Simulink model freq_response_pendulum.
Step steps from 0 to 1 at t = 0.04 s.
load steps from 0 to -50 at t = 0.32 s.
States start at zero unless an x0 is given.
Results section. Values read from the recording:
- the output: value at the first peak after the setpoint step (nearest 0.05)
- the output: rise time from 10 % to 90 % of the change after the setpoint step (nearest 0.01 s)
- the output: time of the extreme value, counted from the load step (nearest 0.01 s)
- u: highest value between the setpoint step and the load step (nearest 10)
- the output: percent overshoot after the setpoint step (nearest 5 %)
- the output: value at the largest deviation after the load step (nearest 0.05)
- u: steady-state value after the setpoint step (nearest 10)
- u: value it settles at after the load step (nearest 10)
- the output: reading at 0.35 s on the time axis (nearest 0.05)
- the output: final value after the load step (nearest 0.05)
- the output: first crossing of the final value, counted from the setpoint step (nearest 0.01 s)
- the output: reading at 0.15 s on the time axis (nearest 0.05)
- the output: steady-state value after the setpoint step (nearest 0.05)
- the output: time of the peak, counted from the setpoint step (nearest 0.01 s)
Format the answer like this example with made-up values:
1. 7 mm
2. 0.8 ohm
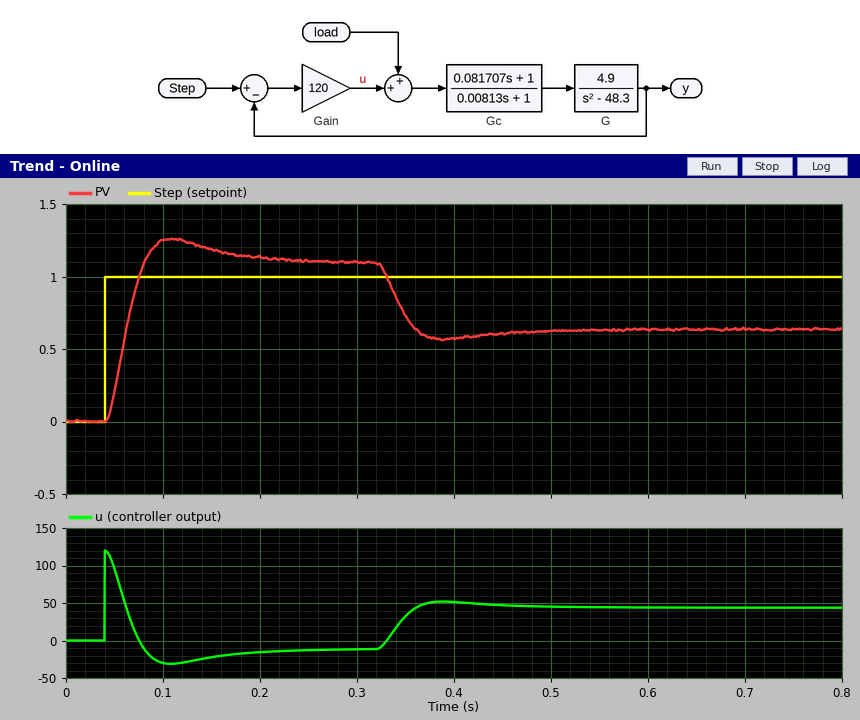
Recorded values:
1. 1.25
2. 0.03 s
3. 0.07 s
4. 120
5. 15 %
6. 0.55
7. -10
8. 40
9. 0.75
10. 0.65
11. 0.04 s
12. 1.20
13. 1.10
14. 0.07 s
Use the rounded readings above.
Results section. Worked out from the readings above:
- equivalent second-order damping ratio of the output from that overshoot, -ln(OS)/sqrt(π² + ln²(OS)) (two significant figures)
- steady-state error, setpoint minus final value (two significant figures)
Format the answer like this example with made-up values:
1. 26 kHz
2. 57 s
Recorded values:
1. 0.52
2. -0.10
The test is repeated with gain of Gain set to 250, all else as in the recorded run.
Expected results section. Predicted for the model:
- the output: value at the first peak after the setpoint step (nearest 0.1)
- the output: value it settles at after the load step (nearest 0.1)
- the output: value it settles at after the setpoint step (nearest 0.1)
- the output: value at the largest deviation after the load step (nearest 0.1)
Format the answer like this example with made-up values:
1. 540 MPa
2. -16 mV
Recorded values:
1. 1.3
2. 0.8
3. 1.0
4. 0.8
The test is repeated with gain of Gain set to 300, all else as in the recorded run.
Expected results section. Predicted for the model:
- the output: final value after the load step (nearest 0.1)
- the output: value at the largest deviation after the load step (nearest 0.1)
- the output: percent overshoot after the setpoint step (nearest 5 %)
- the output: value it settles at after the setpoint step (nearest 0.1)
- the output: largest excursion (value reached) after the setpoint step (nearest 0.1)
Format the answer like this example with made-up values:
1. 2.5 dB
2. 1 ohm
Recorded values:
1. 0.9
2. 0.8
3. 25 %
4. 1.0
5. 1.3
